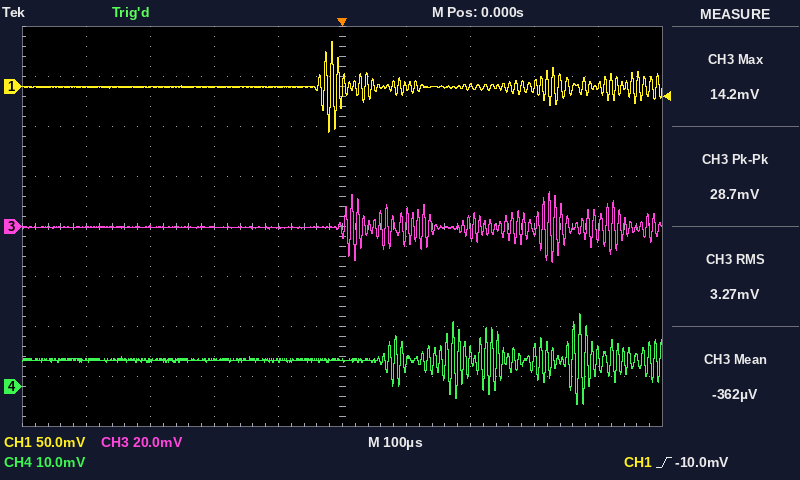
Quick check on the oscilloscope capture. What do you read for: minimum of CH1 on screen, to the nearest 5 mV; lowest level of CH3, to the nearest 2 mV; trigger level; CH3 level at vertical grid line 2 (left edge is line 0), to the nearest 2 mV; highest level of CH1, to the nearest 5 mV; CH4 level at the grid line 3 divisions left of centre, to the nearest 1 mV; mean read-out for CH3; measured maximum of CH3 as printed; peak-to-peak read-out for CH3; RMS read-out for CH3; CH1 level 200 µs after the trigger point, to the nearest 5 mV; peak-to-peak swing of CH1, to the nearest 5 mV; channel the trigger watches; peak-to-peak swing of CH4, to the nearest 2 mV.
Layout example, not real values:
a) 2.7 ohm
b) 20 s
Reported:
a) -45 mV
b) -14 mV
c) -10.0 mV
d) 0 mV
e) 45 mV
f) 5 mV
g) -362 µV
h) 14.2 mV
i) 28.7 mV
j) 3.27 mV
k) 0 mV
l) 90 mV
m) CH1
n) 18 mV
